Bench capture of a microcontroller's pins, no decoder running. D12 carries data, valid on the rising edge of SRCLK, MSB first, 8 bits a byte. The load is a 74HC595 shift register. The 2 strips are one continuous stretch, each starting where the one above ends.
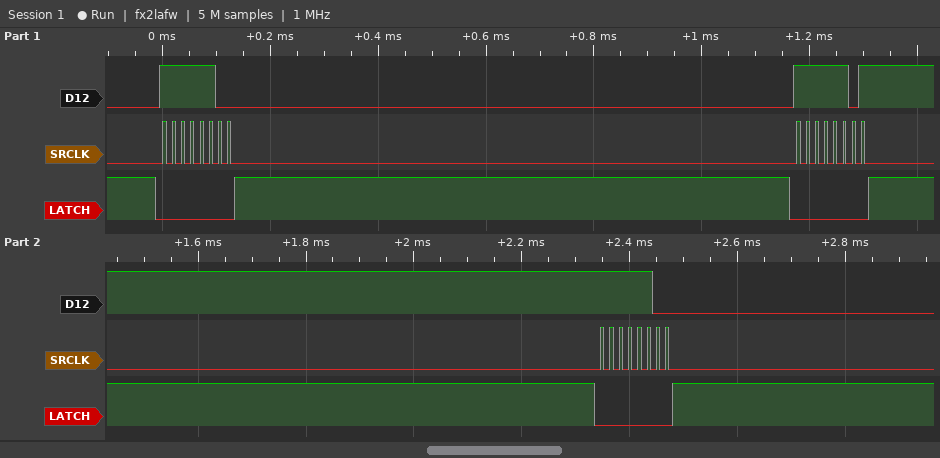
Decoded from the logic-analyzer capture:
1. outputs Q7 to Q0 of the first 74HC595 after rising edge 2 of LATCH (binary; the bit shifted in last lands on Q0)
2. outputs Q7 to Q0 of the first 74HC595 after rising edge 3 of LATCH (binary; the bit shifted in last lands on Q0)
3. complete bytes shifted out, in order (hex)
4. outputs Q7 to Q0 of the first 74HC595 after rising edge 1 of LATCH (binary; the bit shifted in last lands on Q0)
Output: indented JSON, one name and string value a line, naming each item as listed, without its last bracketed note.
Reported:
{
  "outputs Q7 to Q0 of the first 74HC595 after rising edge 2 of LATCH": "11111101",
  "outputs Q7 to Q0 of the first 74HC595 after rising edge 3 of LATCH": "11111100",
  "complete bytes shifted out, in order": "0xFC 0xFD 0xFC",
  "outputs Q7 to Q0 of the first 74HC595 after rising edge 1 of LATCH": "11111100"
}
